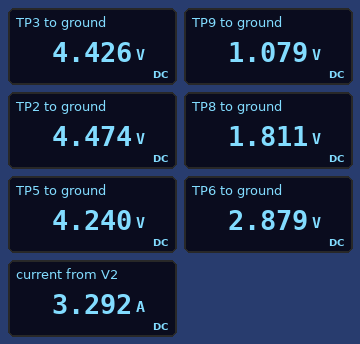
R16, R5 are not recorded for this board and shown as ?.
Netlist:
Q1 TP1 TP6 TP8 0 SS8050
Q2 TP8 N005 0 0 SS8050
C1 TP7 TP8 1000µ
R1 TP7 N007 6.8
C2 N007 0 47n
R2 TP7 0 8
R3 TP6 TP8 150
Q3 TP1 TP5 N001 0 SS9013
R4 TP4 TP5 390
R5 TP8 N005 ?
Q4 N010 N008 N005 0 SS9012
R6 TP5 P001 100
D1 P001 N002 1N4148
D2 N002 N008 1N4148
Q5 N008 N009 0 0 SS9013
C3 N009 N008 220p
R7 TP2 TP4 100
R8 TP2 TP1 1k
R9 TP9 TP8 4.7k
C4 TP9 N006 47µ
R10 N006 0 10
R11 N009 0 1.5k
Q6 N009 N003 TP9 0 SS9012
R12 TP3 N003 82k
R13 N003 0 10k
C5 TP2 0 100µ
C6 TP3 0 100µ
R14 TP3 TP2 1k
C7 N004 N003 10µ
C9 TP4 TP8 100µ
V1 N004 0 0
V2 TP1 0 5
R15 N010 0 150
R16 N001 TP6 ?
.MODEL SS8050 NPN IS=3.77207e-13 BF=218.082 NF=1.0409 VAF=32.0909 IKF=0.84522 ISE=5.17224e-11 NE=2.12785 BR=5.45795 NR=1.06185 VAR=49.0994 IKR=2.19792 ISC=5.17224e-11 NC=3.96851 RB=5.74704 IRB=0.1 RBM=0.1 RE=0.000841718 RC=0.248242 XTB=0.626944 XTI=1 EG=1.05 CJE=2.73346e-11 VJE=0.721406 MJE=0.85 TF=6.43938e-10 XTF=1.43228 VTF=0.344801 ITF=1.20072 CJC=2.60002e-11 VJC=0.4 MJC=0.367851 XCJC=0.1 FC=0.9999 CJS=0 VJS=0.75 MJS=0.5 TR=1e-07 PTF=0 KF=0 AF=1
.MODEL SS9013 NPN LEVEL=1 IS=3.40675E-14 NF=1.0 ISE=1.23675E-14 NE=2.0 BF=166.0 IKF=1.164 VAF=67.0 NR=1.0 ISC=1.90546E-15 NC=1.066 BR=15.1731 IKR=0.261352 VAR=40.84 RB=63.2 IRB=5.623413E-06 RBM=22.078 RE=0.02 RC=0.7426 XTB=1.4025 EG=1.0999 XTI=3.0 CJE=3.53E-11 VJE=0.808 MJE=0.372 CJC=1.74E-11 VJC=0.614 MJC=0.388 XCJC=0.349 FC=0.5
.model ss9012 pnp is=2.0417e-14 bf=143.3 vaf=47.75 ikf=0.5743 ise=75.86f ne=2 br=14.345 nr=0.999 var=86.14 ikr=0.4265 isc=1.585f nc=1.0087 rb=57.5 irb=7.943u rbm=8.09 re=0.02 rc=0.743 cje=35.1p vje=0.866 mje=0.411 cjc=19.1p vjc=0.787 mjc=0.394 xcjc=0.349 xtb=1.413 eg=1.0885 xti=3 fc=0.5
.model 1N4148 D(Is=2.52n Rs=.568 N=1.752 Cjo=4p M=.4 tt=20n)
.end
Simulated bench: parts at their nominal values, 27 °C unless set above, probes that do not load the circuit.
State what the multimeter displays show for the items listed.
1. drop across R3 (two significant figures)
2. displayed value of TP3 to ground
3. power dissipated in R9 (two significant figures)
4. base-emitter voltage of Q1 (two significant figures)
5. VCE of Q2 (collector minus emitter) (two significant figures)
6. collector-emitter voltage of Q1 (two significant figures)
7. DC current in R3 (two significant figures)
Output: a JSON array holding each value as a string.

["1.1 V", "4.426 V", "110 µW", "1.1 V", "1.8 V", "3.2 V", "7.1 mA"]
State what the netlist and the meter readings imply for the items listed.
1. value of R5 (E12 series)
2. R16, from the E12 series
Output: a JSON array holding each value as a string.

["10 Ω", "8.2 Ω"]
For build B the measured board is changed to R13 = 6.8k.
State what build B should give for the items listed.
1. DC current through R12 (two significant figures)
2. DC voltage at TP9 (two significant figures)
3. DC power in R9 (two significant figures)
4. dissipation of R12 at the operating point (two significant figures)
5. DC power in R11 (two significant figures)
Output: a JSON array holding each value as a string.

["50 µA", "940 mV", "160 µW", "200 µW", "51 µW"]
